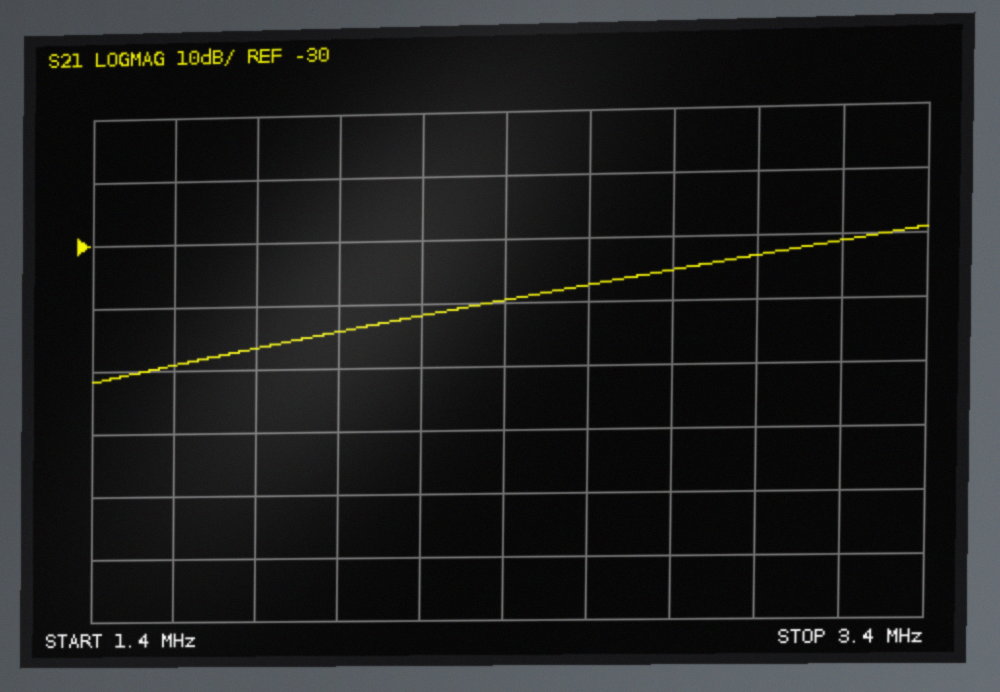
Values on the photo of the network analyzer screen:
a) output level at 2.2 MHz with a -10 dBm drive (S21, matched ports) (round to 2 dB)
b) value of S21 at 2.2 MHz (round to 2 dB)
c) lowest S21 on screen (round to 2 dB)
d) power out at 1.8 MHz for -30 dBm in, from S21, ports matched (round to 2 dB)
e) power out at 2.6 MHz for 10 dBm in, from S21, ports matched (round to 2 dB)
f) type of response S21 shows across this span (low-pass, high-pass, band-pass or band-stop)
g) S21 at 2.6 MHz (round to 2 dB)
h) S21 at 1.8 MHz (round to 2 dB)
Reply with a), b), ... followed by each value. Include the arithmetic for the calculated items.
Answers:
a) -10 dBm + (-42 dB) = -52 dBm
b) -42 dB
c) -52 dB
d) -30 dBm + (-46 dB) = -76 dBm
e) 10 dBm + (-38 dB) = -28 dBm
f) high-pass
g) -38 dB
h) -46 dB
